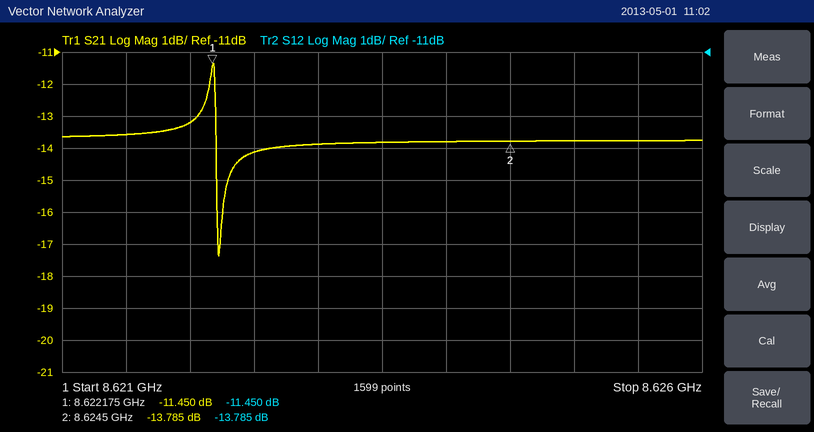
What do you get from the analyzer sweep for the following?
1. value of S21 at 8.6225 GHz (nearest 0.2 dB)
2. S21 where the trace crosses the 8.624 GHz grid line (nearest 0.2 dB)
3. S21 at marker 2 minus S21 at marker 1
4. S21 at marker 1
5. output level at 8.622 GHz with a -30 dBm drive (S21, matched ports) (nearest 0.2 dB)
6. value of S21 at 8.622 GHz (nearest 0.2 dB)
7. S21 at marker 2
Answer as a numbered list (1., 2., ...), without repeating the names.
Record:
1. -14.2 dB
2. -13.8 dB
3. -2.335 dB
4. -11.450 dB
5. -43.2 dBm
6. -13.2 dB
7. -13.785 dB
